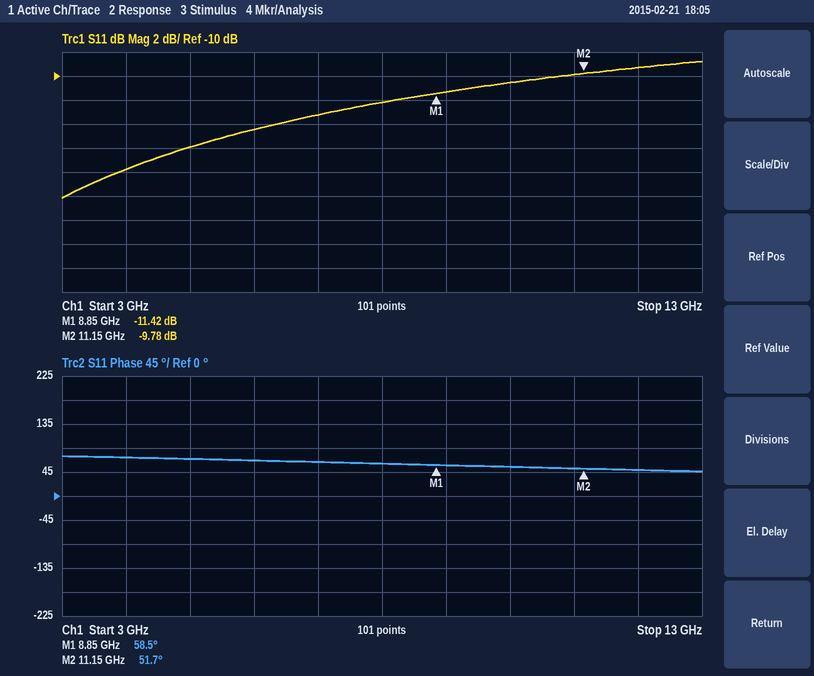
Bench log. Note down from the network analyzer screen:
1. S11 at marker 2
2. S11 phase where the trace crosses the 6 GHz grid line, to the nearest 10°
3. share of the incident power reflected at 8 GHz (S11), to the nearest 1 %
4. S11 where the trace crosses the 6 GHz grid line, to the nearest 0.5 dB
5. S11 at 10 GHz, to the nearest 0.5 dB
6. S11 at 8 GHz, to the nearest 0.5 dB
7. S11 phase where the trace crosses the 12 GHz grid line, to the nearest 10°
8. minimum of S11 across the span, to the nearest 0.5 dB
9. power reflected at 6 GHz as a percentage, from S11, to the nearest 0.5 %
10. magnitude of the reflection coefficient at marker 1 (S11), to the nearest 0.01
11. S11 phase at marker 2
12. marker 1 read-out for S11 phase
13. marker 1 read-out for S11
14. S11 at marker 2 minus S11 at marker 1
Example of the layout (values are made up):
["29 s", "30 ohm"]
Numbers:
["-9.78 dB", "70°", "6 %", "-14.5 dB", "-10.5 dB", "-12.0 dB", "50°", "-20.0 dB", "3.5 %", "0.27", "51.7°", "58.5°", "-11.42 dB", "1.64 dB"]
